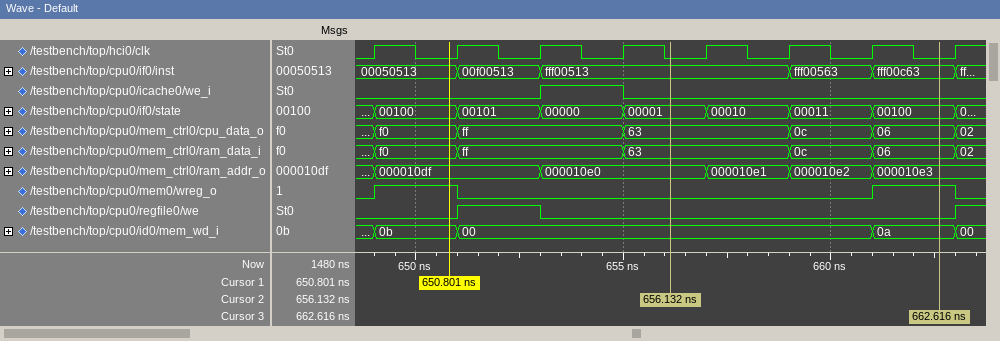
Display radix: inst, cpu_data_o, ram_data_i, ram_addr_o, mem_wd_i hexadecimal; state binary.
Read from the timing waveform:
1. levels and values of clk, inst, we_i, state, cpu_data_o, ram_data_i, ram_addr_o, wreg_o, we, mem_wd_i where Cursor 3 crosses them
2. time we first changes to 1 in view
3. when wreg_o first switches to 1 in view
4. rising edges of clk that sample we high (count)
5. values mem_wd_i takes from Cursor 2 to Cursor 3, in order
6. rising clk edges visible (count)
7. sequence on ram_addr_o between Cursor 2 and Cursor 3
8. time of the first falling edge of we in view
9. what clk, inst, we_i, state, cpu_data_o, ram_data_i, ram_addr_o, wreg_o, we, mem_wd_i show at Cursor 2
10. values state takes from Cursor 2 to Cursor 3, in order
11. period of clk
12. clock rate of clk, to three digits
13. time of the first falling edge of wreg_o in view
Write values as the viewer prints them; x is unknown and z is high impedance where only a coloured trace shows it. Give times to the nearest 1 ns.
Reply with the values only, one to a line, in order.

clk=0, inst=fff00c63, we_i=0, state=00100, cpu_data_o=06, ram_data_i=06, ram_addr_o=000010e3, wreg_o=1, we=0, mem_wd_i=0a
651 ns
649 ns
1
00, 0a
8
000010e0, 000010e1, 000010e2, 000010e3
653 ns
clk=0, inst=fff00513, we_i=0, state=00001, cpu_data_o=63, ram_data_i=63, ram_addr_o=000010e0, wreg_o=0, we=0, mem_wd_i=00
00001, 00010, 00011, 00100
2 ns
500 MHz
651 ns
